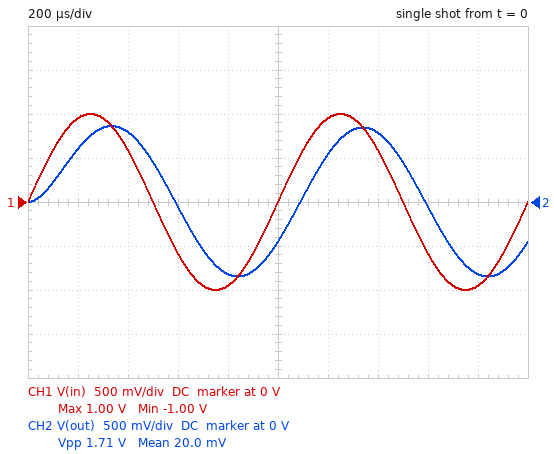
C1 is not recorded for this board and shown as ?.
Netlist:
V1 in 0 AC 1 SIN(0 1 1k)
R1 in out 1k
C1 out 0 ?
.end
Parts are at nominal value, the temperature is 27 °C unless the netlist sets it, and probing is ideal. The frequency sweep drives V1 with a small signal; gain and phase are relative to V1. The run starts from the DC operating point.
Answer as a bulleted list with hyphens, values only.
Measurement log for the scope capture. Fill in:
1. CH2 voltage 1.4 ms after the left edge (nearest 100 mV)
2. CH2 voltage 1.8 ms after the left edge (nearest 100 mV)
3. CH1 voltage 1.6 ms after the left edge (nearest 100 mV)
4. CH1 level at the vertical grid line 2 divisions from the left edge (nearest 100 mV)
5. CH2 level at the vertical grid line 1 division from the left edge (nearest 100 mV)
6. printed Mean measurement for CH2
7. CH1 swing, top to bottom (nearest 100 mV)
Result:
- 800 mV
- -800 mV
- -600 mV
- 600 mV
- 600 mV
- 20.0 mV
- 2.0 V
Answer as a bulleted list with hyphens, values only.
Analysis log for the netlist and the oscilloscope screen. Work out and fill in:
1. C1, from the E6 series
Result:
- 100 nF
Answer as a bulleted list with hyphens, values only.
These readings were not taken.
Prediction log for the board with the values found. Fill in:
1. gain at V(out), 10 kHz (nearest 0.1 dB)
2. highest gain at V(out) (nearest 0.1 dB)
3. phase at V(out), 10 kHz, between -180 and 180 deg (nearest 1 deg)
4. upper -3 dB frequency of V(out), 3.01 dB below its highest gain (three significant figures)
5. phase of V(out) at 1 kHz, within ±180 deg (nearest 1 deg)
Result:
- -16.1 dB
- 0 dB
- -81 deg
- 1.59 kHz
- -32 deg
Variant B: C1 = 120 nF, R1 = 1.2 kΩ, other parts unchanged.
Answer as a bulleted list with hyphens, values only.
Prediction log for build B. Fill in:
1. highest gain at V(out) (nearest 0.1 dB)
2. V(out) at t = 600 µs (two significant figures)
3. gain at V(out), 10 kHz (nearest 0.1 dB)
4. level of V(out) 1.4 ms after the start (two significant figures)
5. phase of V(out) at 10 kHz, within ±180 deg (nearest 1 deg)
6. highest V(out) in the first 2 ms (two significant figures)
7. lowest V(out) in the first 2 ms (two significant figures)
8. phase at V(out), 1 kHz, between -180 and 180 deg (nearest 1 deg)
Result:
- 0 dB
- 87 mV
- -19.2 dB
- 730 mV
- -84 deg
- 780 mV
- -740 mV
- -42 deg
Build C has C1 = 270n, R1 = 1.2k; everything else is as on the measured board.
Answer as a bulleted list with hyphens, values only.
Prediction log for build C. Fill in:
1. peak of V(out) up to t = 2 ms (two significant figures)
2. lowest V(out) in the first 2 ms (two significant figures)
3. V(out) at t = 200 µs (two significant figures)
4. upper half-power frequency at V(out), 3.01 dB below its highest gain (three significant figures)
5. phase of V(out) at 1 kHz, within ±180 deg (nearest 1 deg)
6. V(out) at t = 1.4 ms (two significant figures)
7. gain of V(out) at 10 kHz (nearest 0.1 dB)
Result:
- 550 mV
- -440 mV
- 280 mV
- 491 Hz
- -64 deg
- 440 mV
- -26.2 dB
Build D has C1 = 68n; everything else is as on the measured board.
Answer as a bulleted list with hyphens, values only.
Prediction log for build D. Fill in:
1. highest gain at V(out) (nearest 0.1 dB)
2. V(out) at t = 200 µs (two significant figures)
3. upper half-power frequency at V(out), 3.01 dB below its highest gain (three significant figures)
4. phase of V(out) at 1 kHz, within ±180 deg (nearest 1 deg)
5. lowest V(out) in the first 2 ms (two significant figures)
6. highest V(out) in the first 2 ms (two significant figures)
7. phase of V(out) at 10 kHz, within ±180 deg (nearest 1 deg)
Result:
- 0 dB
- 710 mV
- 2.34 kHz
- -23 deg
- -920 mV
- 920 mV
- -77 deg
